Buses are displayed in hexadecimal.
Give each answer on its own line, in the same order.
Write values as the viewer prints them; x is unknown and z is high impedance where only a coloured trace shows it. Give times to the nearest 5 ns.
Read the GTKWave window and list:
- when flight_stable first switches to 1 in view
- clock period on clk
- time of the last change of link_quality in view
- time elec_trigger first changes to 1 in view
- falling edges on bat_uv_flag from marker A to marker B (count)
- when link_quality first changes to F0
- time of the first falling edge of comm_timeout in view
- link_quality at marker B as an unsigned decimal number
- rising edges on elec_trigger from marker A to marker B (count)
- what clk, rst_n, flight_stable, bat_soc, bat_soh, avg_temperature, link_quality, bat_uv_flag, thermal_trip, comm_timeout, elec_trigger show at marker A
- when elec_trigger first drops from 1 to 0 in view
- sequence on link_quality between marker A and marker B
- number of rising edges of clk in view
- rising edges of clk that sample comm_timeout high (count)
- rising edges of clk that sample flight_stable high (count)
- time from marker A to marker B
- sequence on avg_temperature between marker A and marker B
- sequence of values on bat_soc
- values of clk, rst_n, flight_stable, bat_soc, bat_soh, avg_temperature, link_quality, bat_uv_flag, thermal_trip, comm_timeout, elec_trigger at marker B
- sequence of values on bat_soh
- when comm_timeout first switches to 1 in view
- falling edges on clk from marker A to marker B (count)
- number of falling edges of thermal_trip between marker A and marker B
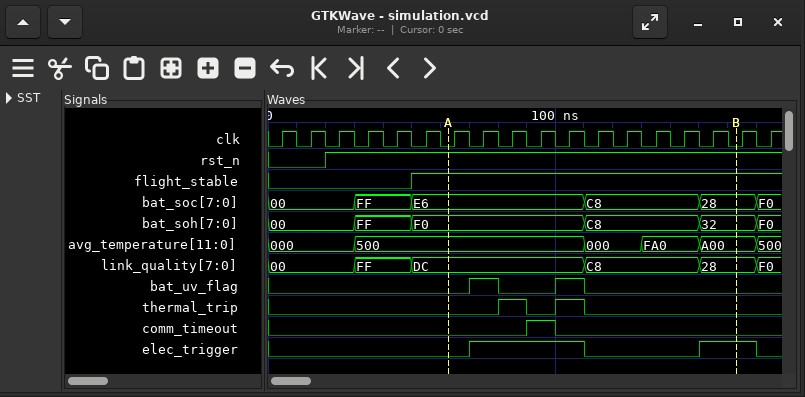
50 ns
10 ns
170 ns
70 ns
2
170 ns
100 ns
40
2
clk=0, rst_n=1, flight_stable=1, bat_soc=E6, bat_soh=F0, avg_temperature=500, link_quality=DC, bat_uv_flag=0, thermal_trip=0, comm_timeout=0, elec_trigger=0
110 ns
DC, C8, 28
18
1
13
100 ns
500, 000, FA0, A00
00, FF, E6, C8, 28, F0
clk=0, rst_n=1, flight_stable=1, bat_soc=28, bat_soh=32, avg_temperature=A00, link_quality=28, bat_uv_flag=0, thermal_trip=0, comm_timeout=0, elec_trigger=1
00, FF, F0, C8, 32, F0
90 ns
10
2
